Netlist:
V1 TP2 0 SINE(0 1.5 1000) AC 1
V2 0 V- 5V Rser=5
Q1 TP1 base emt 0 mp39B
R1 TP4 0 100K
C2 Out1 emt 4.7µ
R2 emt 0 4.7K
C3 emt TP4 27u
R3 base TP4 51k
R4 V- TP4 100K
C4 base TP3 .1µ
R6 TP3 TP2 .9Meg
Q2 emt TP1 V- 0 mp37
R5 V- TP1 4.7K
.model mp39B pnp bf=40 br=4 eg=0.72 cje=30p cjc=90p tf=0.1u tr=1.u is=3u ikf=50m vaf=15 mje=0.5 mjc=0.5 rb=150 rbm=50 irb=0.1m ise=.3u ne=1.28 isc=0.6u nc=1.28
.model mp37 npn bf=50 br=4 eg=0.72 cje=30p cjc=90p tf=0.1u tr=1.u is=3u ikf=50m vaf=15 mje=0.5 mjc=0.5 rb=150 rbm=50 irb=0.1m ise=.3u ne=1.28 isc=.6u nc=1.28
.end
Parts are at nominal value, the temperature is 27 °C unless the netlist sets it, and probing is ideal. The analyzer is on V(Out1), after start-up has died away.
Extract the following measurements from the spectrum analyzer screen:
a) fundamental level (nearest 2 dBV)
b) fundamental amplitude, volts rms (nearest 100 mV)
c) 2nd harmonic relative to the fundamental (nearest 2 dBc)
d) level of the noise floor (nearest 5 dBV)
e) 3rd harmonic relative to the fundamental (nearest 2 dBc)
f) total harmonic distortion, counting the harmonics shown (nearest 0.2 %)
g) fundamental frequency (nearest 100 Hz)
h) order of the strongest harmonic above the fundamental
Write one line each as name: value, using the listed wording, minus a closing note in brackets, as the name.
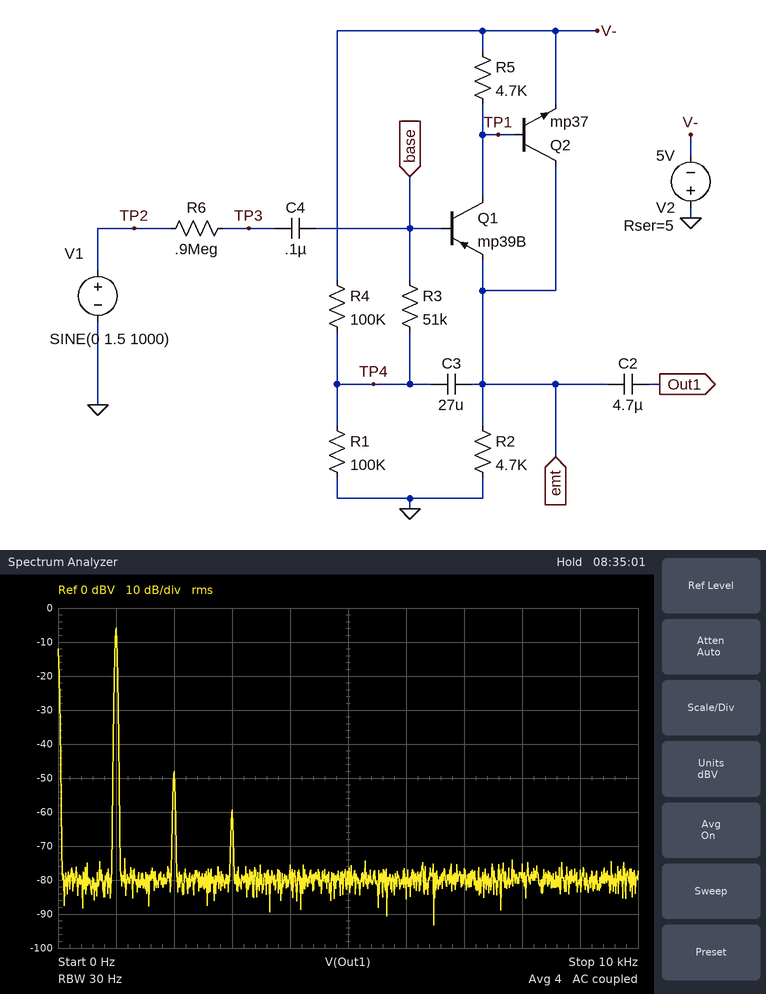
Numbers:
fundamental level: -6 dBV
fundamental amplitude, volts rms: 500 mV
2nd harmonic relative to the fundamental: -42 dBc
level of the noise floor: -80 dBV
3rd harmonic relative to the fundamental: -54 dBc
total harmonic distortion, counting the harmonics shown: 0.8 %
fundamental frequency: 1.0 kHz
order of the strongest harmonic above the fundamental: 2
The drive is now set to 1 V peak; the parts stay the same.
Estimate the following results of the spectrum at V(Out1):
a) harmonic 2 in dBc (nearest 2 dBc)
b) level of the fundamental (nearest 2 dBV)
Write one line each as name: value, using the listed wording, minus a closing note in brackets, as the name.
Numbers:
harmonic 2 in dBc: -46 dBc
level of the fundamental: -10 dBV
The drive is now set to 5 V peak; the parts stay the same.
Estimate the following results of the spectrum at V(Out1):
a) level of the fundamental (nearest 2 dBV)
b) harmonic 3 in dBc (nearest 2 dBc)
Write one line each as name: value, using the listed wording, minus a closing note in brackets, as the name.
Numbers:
level of the fundamental: 4 dBV
harmonic 3 in dBc: -28 dBc
